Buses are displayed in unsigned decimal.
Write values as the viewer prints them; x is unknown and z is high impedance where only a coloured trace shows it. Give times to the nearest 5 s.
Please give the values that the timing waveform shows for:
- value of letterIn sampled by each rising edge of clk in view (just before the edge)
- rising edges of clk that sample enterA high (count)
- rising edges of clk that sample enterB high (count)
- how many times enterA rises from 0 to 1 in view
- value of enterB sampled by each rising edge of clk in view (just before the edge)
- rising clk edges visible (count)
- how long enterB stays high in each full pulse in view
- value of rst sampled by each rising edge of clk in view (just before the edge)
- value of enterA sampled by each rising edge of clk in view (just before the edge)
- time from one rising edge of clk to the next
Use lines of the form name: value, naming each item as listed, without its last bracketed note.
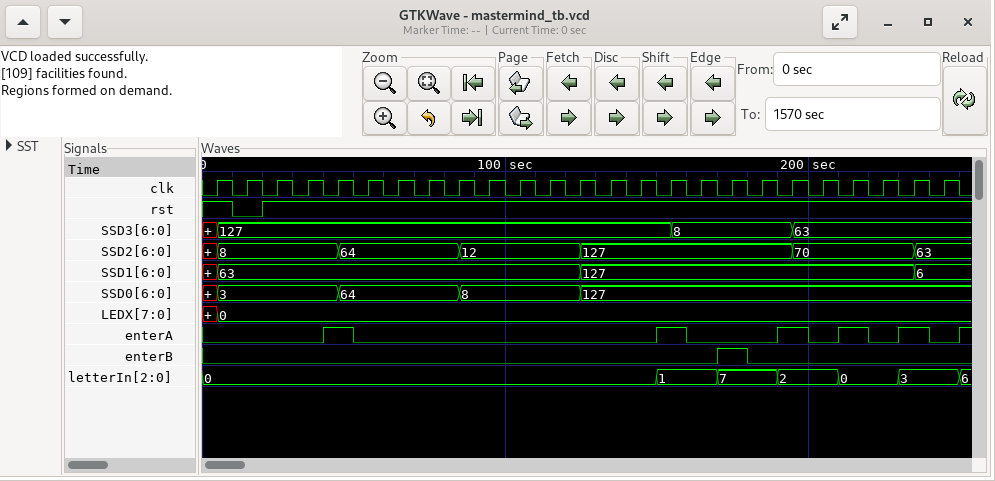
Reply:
value of letterIn sampled by each rising edge of clk in view: 0, 0, 0, 0, 0, 0, 0, 0, 0, 0, 0, 0, 0, 0, 0, 1, 1, 7, 7, 2, 2, 0, 0, 3, 3
rising edges of clk that sample enterA high: 5
rising edges of clk that sample enterB high: 1
how many times enterA rises from 0 to 1 in view: 6
value of enterB sampled by each rising edge of clk in view: 0 0 0 0 0 0 0 0 0 0 0 0 0 0 0 0 0 1 0 0 0 0 0 0 0
rising clk edges visible: 25
how long enterB stays high in each full pulse in view: 10 s
value of rst sampled by each rising edge of clk in view: 1 0 1 1 1 1 1 1 1 1 1 1 1 1 1 1 1 1 1 1 1 1 1 1 1
value of enterA sampled by each rising edge of clk in view: 0 0 0 0 1 0 0 0 0 0 0 0 0 0 0 1 0 0 0 1 0 1 0 1 0
time from one rising edge of clk to the next: 10 s
